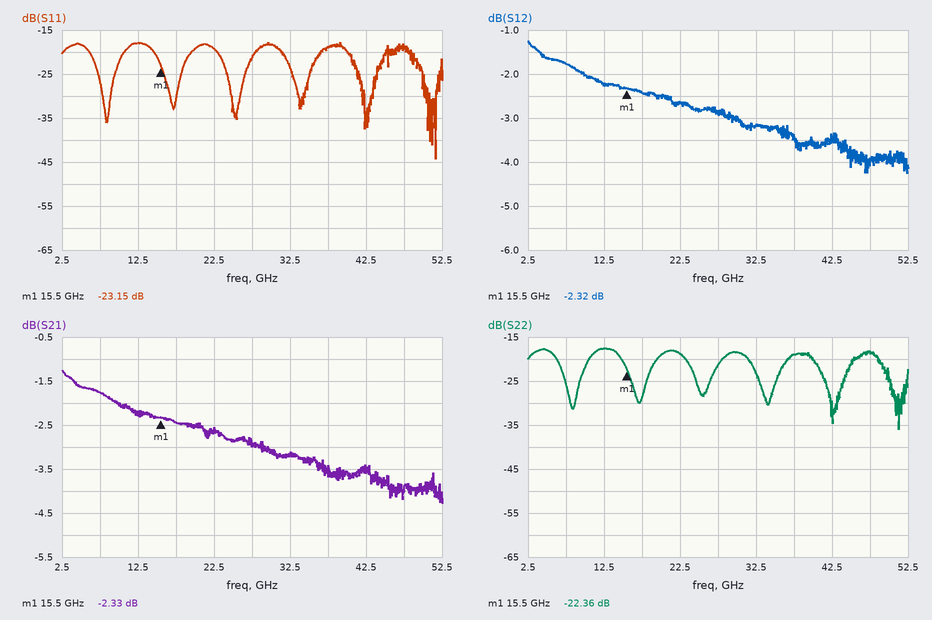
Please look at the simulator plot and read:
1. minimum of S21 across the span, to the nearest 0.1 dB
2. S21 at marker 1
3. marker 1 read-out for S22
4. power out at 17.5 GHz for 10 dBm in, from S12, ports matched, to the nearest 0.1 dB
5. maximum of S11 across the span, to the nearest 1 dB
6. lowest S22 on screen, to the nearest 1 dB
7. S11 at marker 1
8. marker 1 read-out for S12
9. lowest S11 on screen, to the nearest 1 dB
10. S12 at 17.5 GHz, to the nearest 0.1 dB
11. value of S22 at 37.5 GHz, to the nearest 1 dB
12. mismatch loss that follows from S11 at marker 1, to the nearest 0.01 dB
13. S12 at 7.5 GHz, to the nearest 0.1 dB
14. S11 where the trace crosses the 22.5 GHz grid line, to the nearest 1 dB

-4.3 dB
-2.33 dB
-22.36 dB
7.6 dBm
-18 dB
-36 dB
-23.15 dB
-2.32 dB
-44 dB
-2.4 dB
-19 dB
0.02 dB
-1.8 dB
-19 dB
